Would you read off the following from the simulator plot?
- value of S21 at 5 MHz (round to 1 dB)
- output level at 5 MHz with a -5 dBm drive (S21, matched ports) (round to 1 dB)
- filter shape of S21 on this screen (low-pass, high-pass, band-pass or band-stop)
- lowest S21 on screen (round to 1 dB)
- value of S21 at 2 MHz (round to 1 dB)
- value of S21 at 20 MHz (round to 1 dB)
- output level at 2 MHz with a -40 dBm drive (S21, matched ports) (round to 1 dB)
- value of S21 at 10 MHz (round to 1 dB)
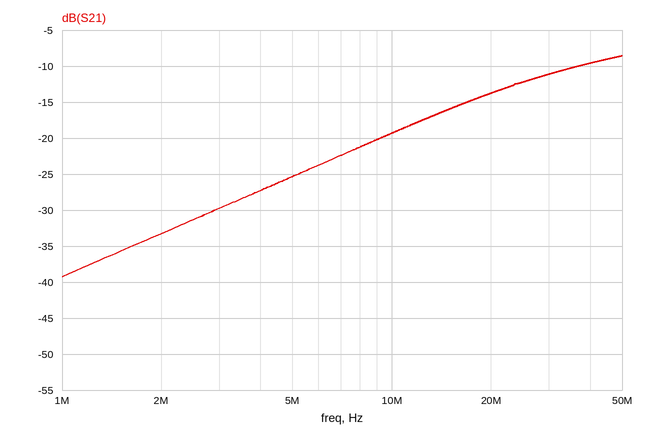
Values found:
-25 dB
-30 dBm
high-pass
-39 dB
-33 dB
-14 dB
-73 dBm
-19 dB
